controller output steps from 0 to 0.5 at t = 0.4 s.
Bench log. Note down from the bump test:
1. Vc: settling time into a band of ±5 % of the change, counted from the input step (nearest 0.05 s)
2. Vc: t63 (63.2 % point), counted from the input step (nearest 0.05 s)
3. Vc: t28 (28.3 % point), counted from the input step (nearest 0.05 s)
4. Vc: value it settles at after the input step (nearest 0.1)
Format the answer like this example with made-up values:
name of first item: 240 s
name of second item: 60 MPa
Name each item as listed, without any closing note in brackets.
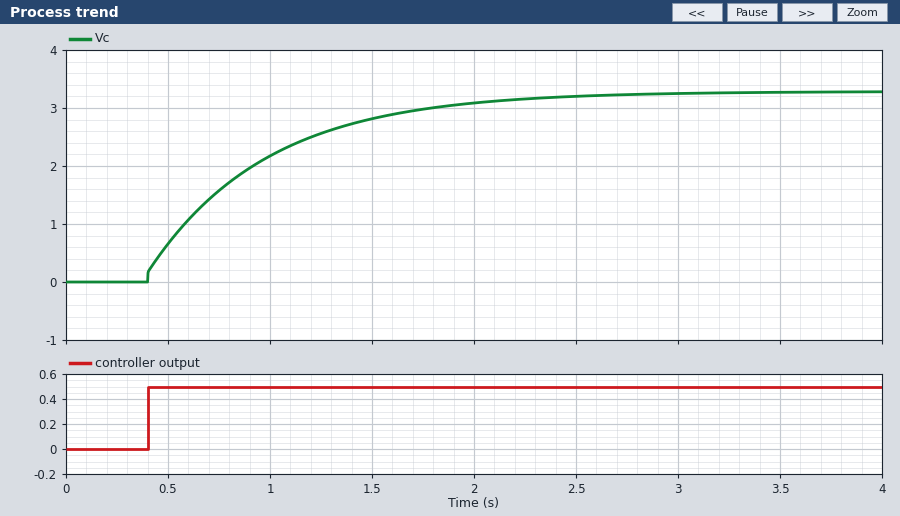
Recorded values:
Vc: settling time into a band of ±5 % of the change, counted from the input step: 1.70 s
Vc: t63 (63.2 % point), counted from the input step: 0.55 s
Vc: t28 (28.3 % point), counted from the input step: 0.15 s
Vc: value it settles at after the input step: 3.3
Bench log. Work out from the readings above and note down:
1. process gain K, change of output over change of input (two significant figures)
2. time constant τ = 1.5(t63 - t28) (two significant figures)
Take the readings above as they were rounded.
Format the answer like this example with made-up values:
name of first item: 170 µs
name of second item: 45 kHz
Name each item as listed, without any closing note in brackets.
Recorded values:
process gain K, change of output over change of input: 6.6
time constant τ = 1.5(t63 - t28): 0.60 s
